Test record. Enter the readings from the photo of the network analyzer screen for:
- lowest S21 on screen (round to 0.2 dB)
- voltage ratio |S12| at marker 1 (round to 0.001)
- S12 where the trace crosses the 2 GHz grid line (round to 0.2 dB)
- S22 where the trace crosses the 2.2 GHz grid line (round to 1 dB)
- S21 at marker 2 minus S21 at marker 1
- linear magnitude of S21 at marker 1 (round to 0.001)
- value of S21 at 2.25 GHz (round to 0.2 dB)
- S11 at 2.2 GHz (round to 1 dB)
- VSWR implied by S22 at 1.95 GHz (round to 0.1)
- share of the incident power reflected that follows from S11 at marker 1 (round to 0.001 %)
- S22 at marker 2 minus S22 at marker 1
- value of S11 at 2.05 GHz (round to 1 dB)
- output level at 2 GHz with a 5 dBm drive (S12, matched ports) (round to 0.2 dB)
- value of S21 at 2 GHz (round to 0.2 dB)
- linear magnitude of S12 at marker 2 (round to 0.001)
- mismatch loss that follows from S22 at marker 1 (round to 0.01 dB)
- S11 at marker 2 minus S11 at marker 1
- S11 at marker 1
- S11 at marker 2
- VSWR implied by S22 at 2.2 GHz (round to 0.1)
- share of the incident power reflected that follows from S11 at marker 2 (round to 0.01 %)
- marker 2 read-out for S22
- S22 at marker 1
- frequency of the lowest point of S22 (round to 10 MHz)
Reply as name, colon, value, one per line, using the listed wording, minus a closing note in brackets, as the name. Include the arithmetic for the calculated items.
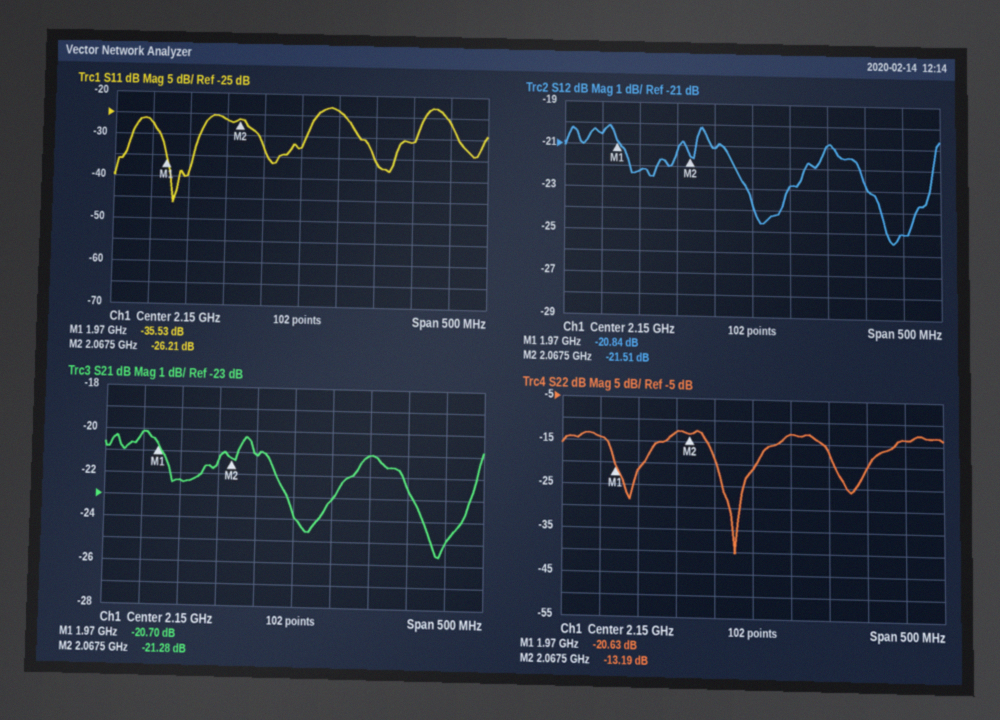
lowest S21 on screen: -25.6 dB
voltage ratio |S12| at marker 1: 10^(-20.84/20) ≈ 0.091
S12 where the trace crosses the 2 GHz grid line: -22.2 dB
S22 where the trace crosses the 2.2 GHz grid line: -13 dB
S21 at marker 2 minus S21 at marker 1: -21.28 − (-20.7) = -0.58 dB
linear magnitude of S21 at marker 1: 10^(-20.7/20) ≈ 0.092
value of S21 at 2.25 GHz: -21.0 dB
S11 at 2.2 GHz: -24 dB
VSWR implied by S22 at 1.95 GHz: |Γ| = 10^(-14/20) = 0.1995; VSWR = (1 + 0.1995)/(1 − 0.1995) ≈ 1.5
share of the incident power reflected that follows from S11 at marker 1: 10^(-35.53/10) ≈ 0.028 %
S22 at marker 2 minus S22 at marker 1: -13.19 − (-20.63) = 7.44 dB
value of S11 at 2.05 GHz: -26 dB
output level at 2 GHz with a 5 dBm drive (S12, matched ports): 5 dBm + (-22.2 dB) = -17.2 dBm
value of S21 at 2 GHz: -22.4 dB
linear magnitude of S12 at marker 2: 10^(-21.51/20) ≈ 0.084
mismatch loss that follows from S22 at marker 1: −10 log10(1 − 10^(-20.63/10)) ≈ 0.04 dB
S11 at marker 2 minus S11 at marker 1: -26.21 − (-35.53) = 9.32 dB
S11 at marker 1: -35.53 dB
S11 at marker 2: -26.21 dB
VSWR implied by S22 at 2.2 GHz: |Γ| = 10^(-13/20) = 0.2239; VSWR = (1 + 0.2239)/(1 − 0.2239) ≈ 1.6
share of the incident power reflected that follows from S11 at marker 2: 10^(-26.21/10) ≈ 0.24 %
marker 2 read-out for S22: -13.19 dB
S22 at marker 1: -20.63 dB
frequency of the lowest point of S22: 2.13 GHz
